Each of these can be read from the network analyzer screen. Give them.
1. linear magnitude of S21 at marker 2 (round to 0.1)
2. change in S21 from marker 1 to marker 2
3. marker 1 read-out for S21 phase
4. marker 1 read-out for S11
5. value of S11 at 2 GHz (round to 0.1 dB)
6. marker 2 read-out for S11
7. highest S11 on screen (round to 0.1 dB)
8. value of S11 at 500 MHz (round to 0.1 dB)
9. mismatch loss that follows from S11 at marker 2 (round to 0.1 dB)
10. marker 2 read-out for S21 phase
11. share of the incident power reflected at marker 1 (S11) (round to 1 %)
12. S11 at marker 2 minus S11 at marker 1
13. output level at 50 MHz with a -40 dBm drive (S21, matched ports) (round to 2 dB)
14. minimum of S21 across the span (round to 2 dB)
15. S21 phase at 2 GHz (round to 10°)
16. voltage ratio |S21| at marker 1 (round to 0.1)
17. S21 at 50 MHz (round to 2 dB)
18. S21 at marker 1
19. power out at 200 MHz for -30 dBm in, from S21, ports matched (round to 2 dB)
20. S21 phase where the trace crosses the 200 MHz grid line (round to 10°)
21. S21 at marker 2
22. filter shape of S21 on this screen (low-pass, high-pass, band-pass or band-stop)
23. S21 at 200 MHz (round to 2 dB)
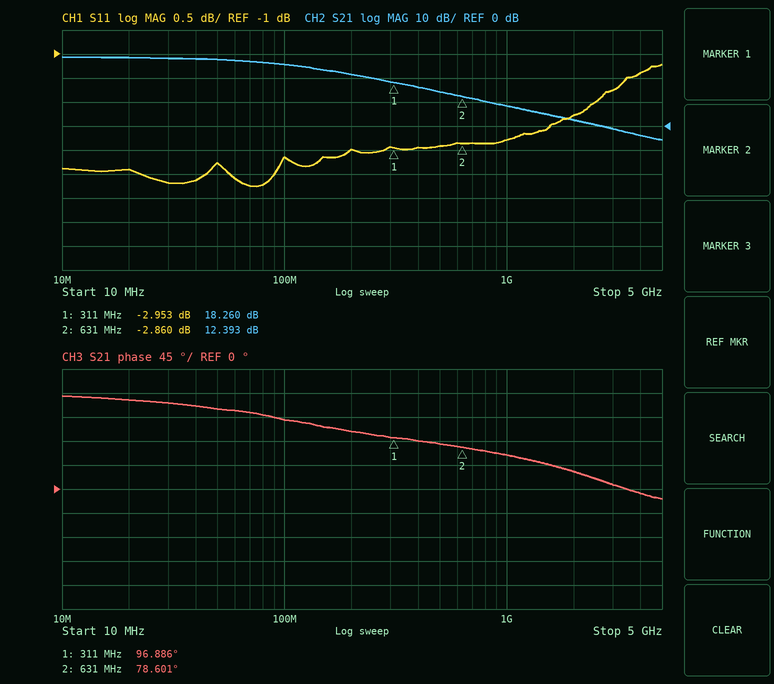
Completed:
4.2
-5.867 dB
96.886°
-2.953 dB
-2.3 dB
-2.860 dB
-1.2 dB
-2.9 dB
3.2 dB
78.601°
51 %
0.093 dB
-12 dBm
-6 dB
30°
8.2
28 dB
18.260 dB
-8 dBm
110°
12.393 dB
low-pass
22 dB
